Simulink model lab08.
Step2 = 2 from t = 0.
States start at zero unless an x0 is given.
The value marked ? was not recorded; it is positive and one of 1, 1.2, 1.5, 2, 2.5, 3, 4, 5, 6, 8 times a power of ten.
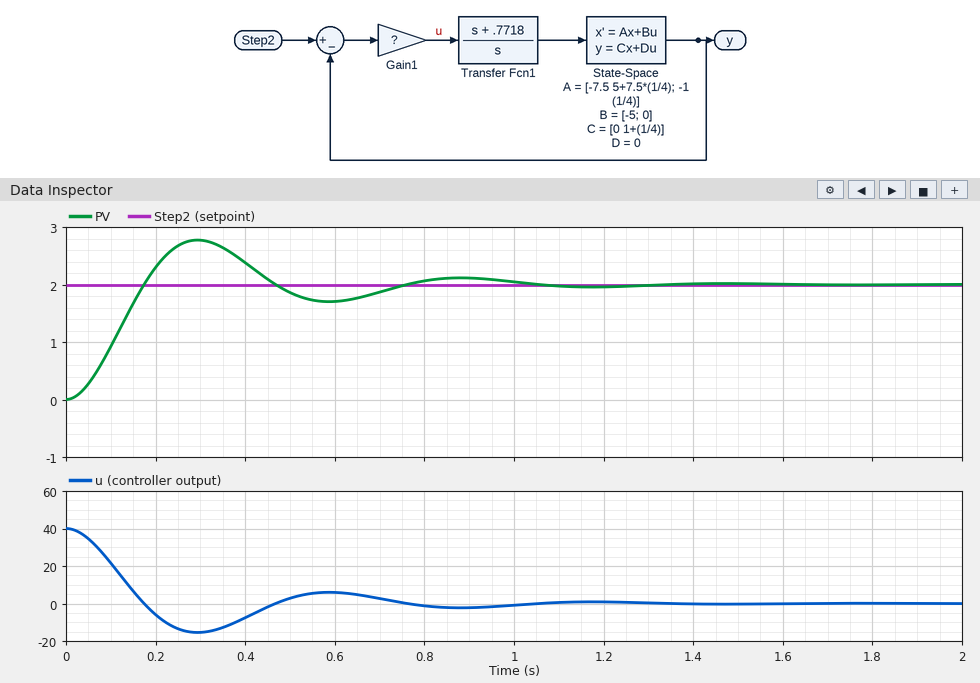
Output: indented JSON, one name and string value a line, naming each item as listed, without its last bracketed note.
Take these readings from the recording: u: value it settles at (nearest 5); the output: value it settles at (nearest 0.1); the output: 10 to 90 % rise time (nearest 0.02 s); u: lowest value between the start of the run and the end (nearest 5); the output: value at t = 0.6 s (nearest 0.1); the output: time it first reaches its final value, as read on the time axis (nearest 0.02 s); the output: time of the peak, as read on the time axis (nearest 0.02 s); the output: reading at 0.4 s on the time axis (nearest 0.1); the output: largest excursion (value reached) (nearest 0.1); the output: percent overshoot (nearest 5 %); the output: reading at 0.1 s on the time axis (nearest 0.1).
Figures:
{
  "u: value it settles at": "0",
  "the output: value it settles at": "2.0",
  "the output: 10 to 90 % rise time": "0.12 s",
  "u: lowest value between the start of the run and the end": "-15",
  "the output: value at t = 0.6 s": "1.7",
  "the output: time it first reaches its final value, as read on the time axis": "0.18 s",
  "the output: time of the peak, as read on the time axis": "0.30 s",
  "the output: reading at 0.4 s on the time axis": "2.4",
  "the output: largest excursion (value reached)": "2.8",
  "the output: percent overshoot": "40 %",
  "the output: reading at 0.1 s on the time axis": "0.9"
}
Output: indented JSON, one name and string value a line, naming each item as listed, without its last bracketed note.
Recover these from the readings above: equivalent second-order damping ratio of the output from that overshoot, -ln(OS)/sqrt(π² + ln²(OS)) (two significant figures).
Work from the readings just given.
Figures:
{
  "equivalent second-order damping ratio of the output from that overshoot, -ln(OS)/sqrt(π² + ln²(OS))": "0.28"
}
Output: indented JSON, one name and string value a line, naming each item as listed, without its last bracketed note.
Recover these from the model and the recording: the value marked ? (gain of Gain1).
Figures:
{
  "the value marked ?": "20"
}
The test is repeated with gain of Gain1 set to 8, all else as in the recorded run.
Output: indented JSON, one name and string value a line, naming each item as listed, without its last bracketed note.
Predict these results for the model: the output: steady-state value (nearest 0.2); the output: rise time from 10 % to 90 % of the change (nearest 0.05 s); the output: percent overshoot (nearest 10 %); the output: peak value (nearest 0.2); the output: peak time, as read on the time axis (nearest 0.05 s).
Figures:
{
  "the output: steady-state value": "2.0",
  "the output: rise time from 10 % to 90 % of the change": "0.20 s",
  "the output: percent overshoot": "20 %",
  "the output: peak value": "2.4",
  "the output: peak time, as read on the time axis": "0.50 s"
}
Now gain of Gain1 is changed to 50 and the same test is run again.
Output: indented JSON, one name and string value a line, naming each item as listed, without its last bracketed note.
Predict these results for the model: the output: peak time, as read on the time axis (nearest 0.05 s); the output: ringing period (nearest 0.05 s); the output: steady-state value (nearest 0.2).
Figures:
{
  "the output: peak time, as read on the time axis": "0.20 s",
  "the output: ringing period": "0.35 s",
  "the output: steady-state value": "2.0"
}
